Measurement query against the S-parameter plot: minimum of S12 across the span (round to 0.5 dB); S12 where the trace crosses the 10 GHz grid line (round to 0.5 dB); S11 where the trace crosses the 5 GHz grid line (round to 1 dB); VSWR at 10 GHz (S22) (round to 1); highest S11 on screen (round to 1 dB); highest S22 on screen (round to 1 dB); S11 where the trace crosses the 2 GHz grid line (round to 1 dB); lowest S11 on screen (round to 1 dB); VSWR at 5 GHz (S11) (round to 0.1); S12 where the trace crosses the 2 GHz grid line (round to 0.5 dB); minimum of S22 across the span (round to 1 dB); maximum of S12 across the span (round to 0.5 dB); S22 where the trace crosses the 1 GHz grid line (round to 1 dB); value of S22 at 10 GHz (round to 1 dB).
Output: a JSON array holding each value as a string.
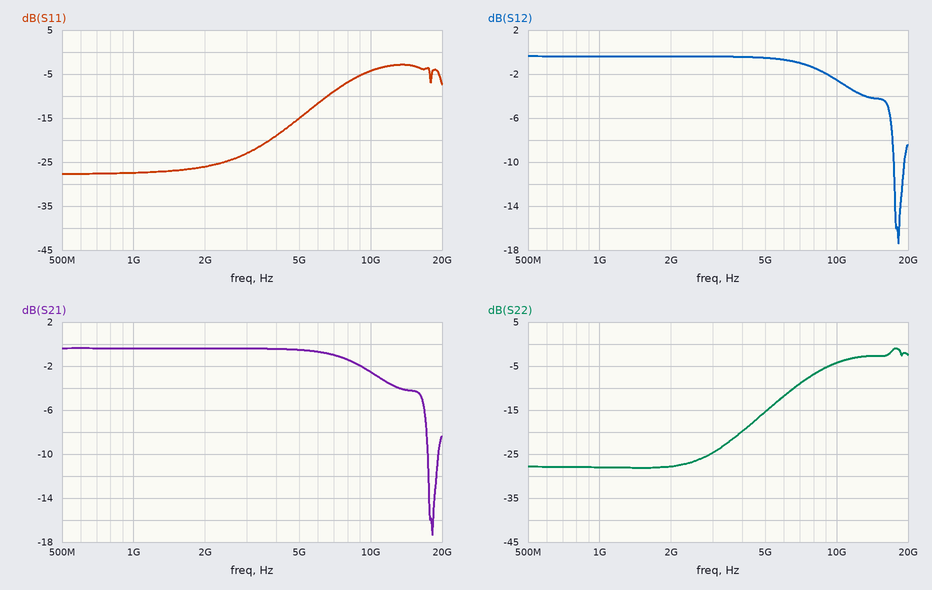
["-17.5 dB", "-2.5 dB", "-15 dB", "4", "-3 dB", "-1 dB", "-26 dB", "-28 dB", "1.4", "-0.5 dB", "-28 dB", "-0.5 dB", "-28 dB", "-4 dB"]
